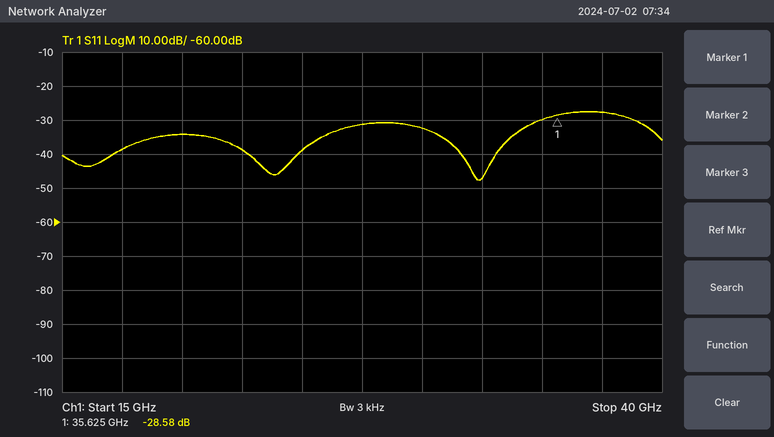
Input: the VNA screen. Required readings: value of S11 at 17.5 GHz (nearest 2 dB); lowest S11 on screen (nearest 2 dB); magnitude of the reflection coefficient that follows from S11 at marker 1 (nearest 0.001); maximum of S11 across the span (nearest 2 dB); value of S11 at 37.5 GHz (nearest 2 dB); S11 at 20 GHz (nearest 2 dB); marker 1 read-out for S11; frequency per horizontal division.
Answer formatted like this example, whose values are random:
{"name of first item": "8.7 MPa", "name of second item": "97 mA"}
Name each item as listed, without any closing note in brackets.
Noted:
{"value of S11 at 17.5 GHz": "-38 dB", "lowest S11 on screen": "-48 dB", "magnitude of the reflection coefficient that follows from S11 at marker 1": "0.037", "maximum of S11 across the span": "-28 dB", "value of S11 at 37.5 GHz": "-28 dB", "S11 at 20 GHz": "-34 dB", "marker 1 read-out for S11": "-28.58 dB", "frequency per horizontal division": "2.5 GHz"}
